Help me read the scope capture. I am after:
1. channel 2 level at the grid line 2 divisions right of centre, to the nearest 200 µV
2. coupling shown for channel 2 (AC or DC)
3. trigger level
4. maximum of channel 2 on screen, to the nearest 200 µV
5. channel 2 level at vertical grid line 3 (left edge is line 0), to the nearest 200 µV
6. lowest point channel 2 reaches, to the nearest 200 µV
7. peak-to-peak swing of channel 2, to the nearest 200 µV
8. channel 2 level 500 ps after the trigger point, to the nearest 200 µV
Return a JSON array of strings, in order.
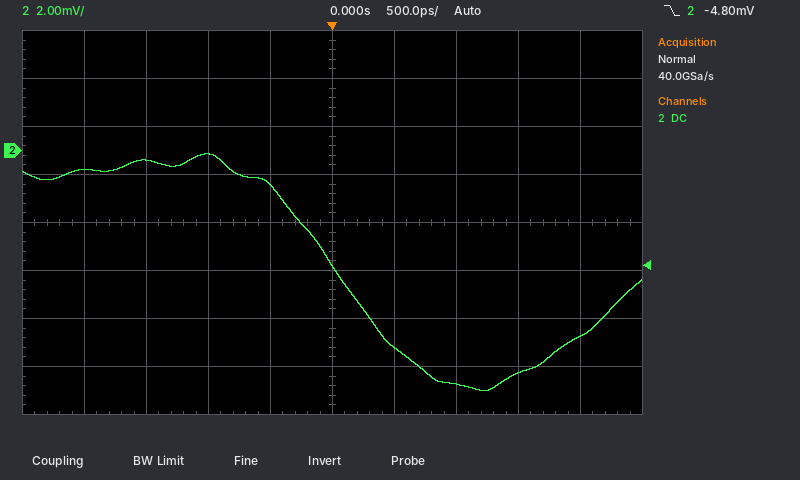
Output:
["-9.8 mV", "DC", "-4.80 mV", "-200 µV", "-200 µV", "-10.0 mV", "9.8 mV", "-8.2 mV"]
